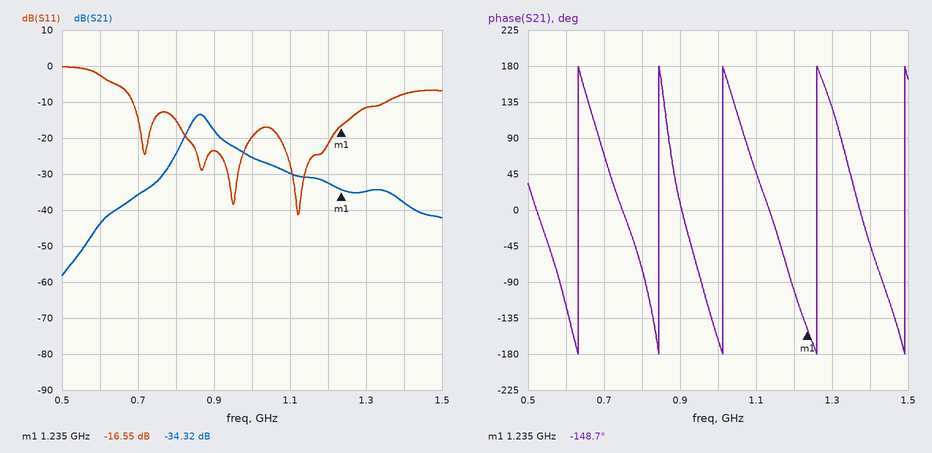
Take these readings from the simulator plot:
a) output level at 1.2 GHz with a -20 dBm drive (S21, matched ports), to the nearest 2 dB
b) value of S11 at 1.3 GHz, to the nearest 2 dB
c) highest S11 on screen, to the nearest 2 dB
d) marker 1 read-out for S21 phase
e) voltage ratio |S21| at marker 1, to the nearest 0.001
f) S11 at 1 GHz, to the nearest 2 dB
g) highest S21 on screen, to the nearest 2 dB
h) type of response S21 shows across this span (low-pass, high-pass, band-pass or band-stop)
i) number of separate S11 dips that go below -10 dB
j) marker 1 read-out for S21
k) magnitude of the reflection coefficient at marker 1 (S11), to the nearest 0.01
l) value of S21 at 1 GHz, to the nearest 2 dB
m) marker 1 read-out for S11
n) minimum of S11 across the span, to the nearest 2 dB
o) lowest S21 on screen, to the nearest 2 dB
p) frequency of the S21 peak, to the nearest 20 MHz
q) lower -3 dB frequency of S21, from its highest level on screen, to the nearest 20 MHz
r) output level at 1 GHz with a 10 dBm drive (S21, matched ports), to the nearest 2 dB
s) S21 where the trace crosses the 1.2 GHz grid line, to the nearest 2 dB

-52 dBm
-12 dB
0 dB
-148.7°
0.019
-20 dB
-14 dB
band-pass
4
-34.32 dB
0.15
-26 dB
-16.55 dB
-42 dB
-58 dB
860 MHz
840 MHz
-16 dBm
-32 dB
